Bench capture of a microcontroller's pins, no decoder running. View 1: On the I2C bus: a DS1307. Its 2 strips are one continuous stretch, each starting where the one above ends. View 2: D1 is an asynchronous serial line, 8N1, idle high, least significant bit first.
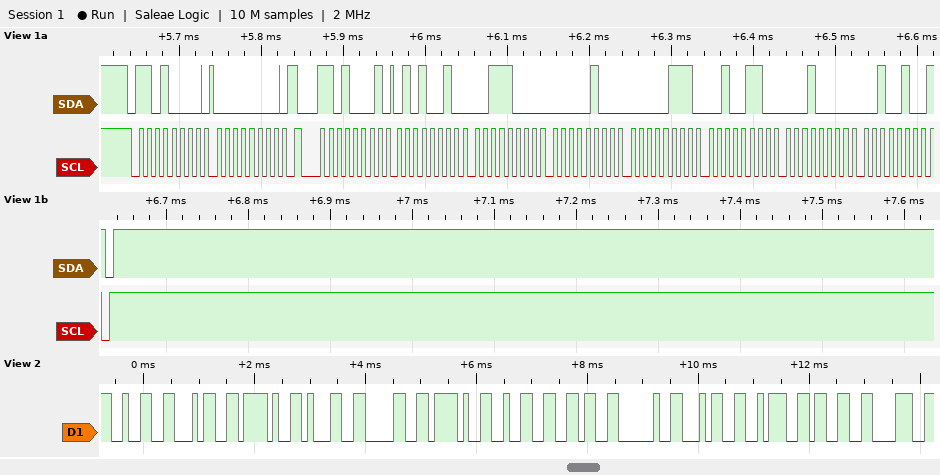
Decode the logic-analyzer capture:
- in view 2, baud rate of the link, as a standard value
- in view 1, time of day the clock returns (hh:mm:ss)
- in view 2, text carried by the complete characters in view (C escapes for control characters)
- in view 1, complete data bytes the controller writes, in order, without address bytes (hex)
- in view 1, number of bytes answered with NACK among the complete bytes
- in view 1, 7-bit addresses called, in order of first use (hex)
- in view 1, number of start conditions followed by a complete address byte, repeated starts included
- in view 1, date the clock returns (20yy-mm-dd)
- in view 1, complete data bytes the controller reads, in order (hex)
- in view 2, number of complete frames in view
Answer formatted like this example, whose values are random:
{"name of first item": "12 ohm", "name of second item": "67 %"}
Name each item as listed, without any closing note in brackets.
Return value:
{"in view 2, baud rate of the link, as a standard value": "9600 baud", "in view 1, time of day the clock returns": "04:38:52", "in view 2, text carried by the complete characters in view": "\"24/10/26 4:38\"", "in view 1, complete data bytes the controller writes, in order, without address bytes": "00", "in view 1, number of bytes answered with NACK among the complete bytes": "1", "in view 1, 7-bit addresses called, in order of first use": "0x68", "in view 1, number of start conditions followed by a complete address byte, repeated starts included": "2", "in view 1, date the clock returns": "2024-10-26", "in view 1, complete data bytes the controller reads, in order": "52 38 04 07 26 10 24", "in view 2, number of complete frames in view": "13"}
